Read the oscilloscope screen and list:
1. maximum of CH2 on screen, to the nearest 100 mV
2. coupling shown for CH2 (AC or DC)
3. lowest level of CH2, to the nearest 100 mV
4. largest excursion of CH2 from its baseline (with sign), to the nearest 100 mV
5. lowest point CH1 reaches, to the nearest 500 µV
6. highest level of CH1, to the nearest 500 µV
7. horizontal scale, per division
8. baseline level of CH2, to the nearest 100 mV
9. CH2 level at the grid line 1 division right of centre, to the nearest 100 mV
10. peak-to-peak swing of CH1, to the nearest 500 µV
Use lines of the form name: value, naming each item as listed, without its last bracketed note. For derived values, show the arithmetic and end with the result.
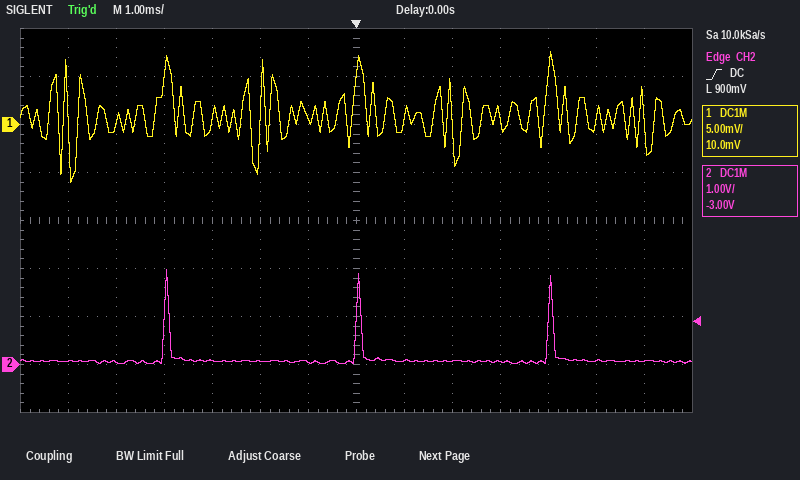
maximum of CH2 on screen, to the nearest 100 mV: 2.0 V
coupling shown for CH2: DC
lowest level of CH2, to the nearest 100 mV: 0.0 V
largest excursion of CH2 from its baseline (with sign), to the nearest 100 mV: 2.0 V − (100 mV) = +1.9 V
lowest point CH1 reaches, to the nearest 500 µV: -6.0 mV
highest level of CH1, to the nearest 500 µV: 7.5 mV
horizontal scale, per division: 1 ms
baseline level of CH2, to the nearest 100 mV: 100 mV
CH2 level at the grid line 1 division right of centre, to the nearest 100 mV: 100 mV
peak-to-peak swing of CH1, to the nearest 500 µV: 7.5 mV − (-6.0 mV) = 13.5 mV
